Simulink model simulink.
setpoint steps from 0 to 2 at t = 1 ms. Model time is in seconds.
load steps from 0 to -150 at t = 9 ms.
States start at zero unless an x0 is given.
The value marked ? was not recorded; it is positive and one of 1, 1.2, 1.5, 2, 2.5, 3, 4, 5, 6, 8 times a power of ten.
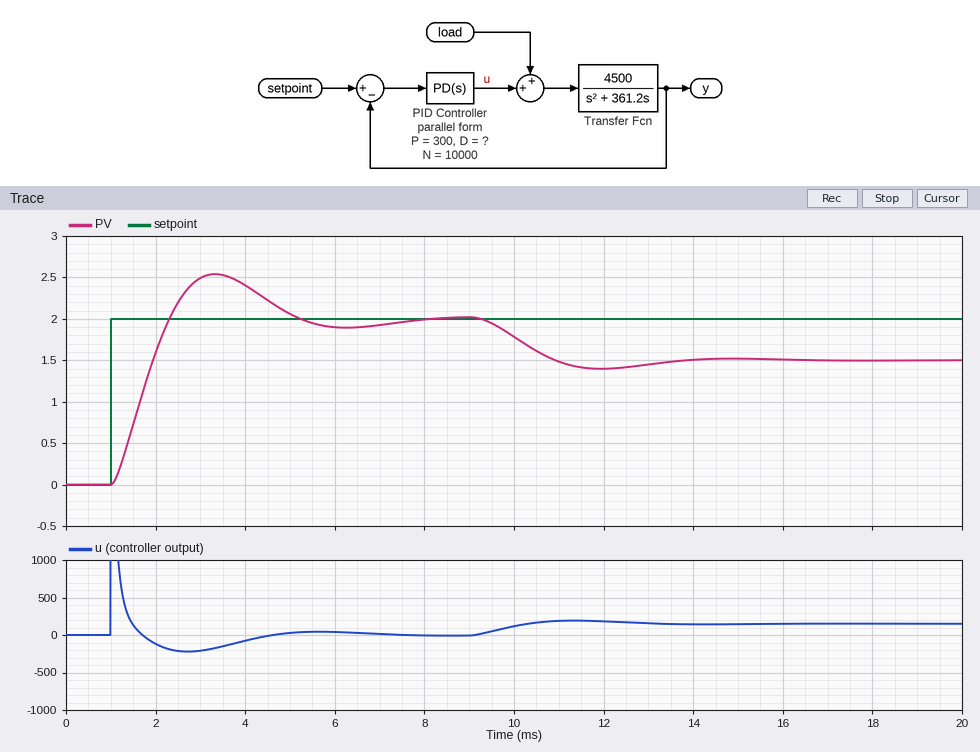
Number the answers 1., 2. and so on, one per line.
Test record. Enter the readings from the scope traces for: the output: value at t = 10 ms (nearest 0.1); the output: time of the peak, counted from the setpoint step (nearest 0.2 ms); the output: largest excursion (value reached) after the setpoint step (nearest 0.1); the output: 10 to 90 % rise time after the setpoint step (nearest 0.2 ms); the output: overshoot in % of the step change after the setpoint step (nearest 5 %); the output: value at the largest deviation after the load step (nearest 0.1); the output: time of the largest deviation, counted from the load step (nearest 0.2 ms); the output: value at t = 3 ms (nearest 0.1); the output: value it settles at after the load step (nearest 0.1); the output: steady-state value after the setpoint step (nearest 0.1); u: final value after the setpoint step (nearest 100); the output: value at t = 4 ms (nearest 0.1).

1. 1.8
2. 2.4 ms
3. 2.5
4. 1.0 ms
5. 25 %
6. 1.4
7. 3.0 ms
8. 2.5
9. 1.5
10. 2.0
11. 0
12. 2.4
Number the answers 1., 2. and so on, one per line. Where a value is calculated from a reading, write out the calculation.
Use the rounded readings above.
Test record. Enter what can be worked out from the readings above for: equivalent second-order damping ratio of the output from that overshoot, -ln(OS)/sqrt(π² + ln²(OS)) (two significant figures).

1. ln(0.25) = -1.386; 1.386 / sqrt(9.870 + 1.922) = 0.40
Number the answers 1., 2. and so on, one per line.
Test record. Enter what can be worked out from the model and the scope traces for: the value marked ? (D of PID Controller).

1. 0.15
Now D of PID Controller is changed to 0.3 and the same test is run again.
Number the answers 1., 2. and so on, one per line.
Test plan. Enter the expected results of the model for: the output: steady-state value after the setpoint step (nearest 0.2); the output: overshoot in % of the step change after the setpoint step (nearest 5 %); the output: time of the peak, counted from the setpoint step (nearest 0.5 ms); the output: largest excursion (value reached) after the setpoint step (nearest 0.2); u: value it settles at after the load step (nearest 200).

1. 2.0
2. 15 %
3. 2.0 ms
4. 2.2
5. 200
